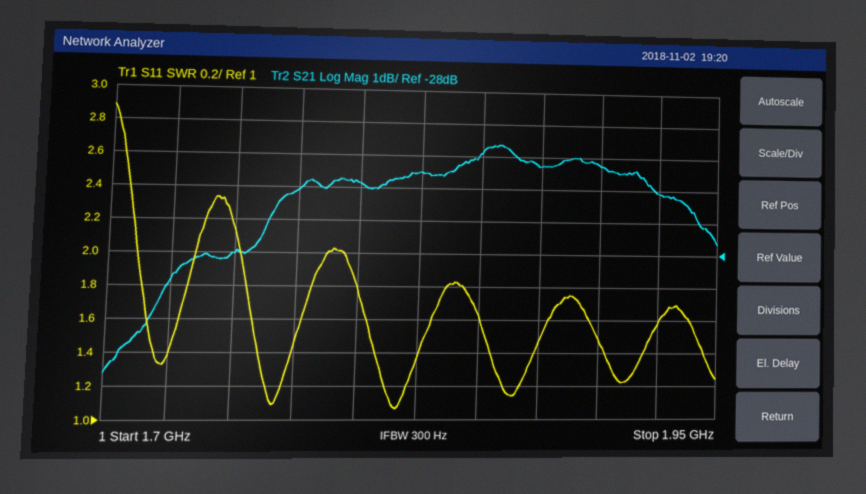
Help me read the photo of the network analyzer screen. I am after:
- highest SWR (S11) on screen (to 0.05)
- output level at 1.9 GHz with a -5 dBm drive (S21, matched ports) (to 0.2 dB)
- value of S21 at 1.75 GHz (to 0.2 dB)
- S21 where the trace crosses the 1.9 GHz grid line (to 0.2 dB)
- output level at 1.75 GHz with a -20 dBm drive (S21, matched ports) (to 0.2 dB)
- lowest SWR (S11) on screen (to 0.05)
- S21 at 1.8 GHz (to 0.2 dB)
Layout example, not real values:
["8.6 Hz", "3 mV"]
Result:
["2.90", "-30.2 dBm", "-28.0 dB", "-25.2 dB", "-48.0 dBm", "1.05", "-25.8 dB"]
